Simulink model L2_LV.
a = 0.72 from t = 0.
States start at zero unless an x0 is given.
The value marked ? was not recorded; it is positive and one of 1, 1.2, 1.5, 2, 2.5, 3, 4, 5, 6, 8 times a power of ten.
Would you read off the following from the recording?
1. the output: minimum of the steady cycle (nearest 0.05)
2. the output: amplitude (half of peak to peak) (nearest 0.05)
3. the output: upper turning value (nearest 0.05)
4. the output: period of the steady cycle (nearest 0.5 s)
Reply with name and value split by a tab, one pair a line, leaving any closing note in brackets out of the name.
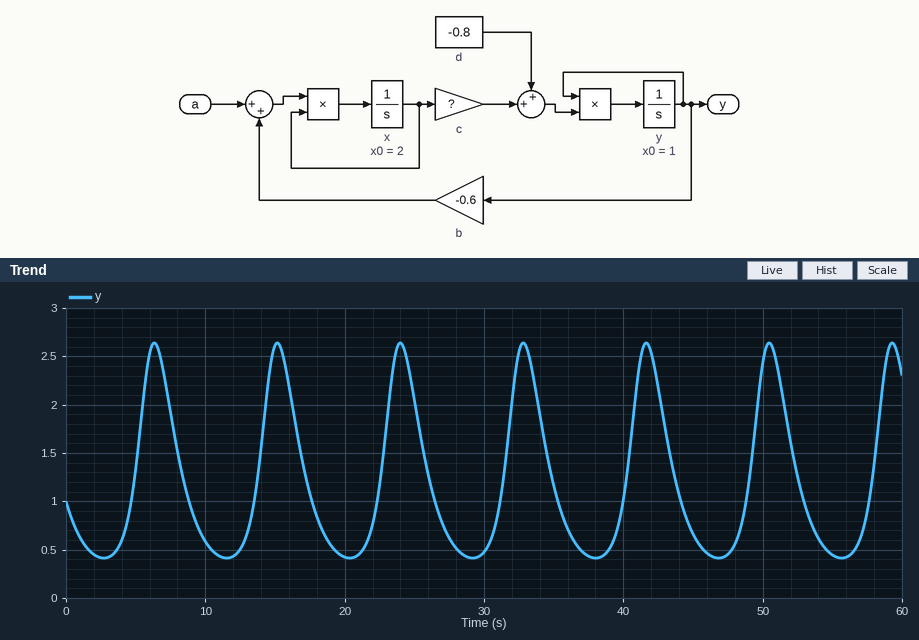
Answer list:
the output: minimum of the steady cycle	0.40
the output: amplitude (half of peak to peak)	1.10
the output: upper turning value	2.65
the output: period of the steady cycle	9.0 s
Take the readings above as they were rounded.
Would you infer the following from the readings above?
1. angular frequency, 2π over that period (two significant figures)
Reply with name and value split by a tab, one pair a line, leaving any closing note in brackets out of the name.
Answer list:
angular frequency, 2π over that period	0.70 rad/s
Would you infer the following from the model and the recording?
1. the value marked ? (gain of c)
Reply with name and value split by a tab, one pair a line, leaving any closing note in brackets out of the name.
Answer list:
the value marked ?	0.15
